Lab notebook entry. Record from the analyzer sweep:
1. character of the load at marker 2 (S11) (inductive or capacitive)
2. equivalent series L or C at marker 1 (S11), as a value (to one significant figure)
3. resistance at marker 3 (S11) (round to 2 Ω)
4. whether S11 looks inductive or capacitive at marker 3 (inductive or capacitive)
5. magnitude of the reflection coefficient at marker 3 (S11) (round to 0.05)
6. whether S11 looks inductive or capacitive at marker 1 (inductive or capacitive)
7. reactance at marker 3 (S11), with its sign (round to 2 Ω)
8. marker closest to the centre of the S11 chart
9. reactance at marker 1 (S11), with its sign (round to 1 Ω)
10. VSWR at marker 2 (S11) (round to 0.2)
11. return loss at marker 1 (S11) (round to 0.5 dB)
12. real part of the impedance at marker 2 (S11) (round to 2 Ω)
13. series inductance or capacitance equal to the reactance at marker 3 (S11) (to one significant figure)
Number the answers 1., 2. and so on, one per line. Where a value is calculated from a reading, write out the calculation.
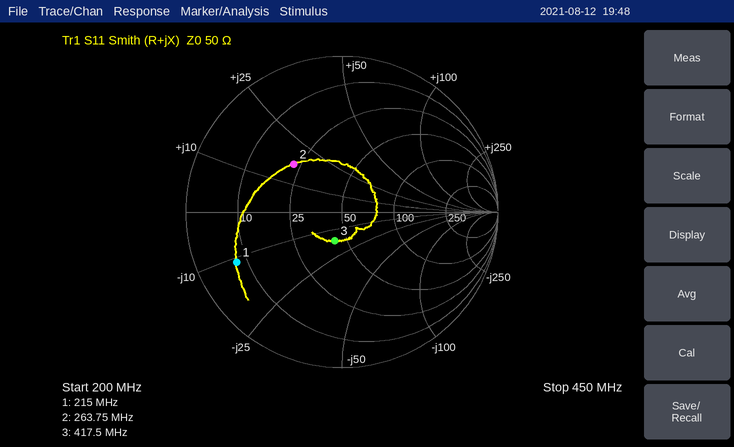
1. inductive
2. C = 1/(2π × 215 MHz × 11 Ω) ≈ 67.3 pF, so 70 pF to one significant figure
3. 42 Ω
4. capacitive
5. 0.20
6. capacitive
7. -16 Ω
8. marker 3
9. -11 Ω
10. 2.6
11. 2.5 dB
12. 22 Ω
13. C = 1/(2π × 417.5 MHz × 16 Ω) ≈ 23.8 pF, so 20 pF to one significant figure
